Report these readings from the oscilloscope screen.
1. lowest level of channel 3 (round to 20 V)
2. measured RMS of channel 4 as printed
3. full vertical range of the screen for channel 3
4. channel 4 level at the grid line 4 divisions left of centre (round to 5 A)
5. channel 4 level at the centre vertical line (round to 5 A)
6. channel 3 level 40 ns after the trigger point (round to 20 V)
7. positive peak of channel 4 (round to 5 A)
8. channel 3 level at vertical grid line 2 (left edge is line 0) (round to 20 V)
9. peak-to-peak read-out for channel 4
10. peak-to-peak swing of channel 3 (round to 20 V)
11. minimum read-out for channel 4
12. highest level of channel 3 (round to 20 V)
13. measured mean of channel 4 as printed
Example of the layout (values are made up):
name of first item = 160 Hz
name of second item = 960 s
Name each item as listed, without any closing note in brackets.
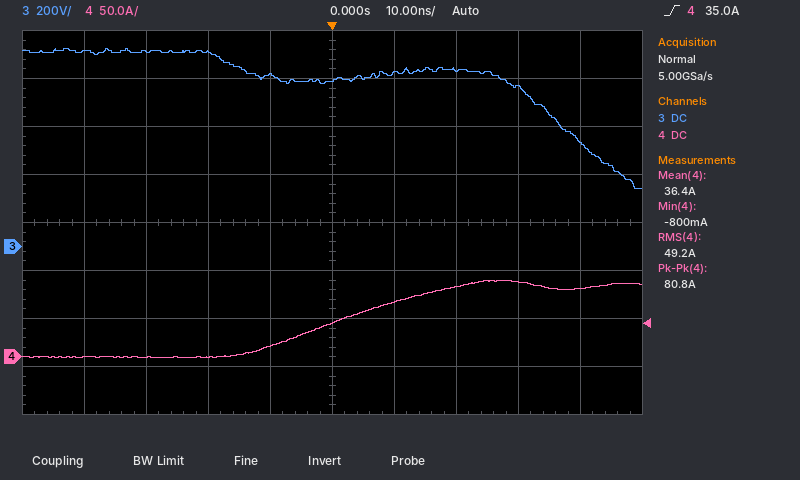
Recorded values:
lowest level of channel 3 = 240 V
measured RMS of channel 4 as printed = 49.2 A
full vertical range of the screen for channel 3 = 1.6 kV
channel 4 level at the grid line 4 divisions left of centre = 0 A
channel 4 level at the centre vertical line = 35 A
channel 3 level 40 ns after the trigger point = 440 V
positive peak of channel 4 = 80 A
channel 3 level at vertical grid line 2 (left edge is line 0) = 820 V
peak-to-peak read-out for channel 4 = 80.8 A
peak-to-peak swing of channel 3 = 580 V
minimum read-out for channel 4 = -800 mA
highest level of channel 3 = 820 V
measured mean of channel 4 as printed = 36.4 A
